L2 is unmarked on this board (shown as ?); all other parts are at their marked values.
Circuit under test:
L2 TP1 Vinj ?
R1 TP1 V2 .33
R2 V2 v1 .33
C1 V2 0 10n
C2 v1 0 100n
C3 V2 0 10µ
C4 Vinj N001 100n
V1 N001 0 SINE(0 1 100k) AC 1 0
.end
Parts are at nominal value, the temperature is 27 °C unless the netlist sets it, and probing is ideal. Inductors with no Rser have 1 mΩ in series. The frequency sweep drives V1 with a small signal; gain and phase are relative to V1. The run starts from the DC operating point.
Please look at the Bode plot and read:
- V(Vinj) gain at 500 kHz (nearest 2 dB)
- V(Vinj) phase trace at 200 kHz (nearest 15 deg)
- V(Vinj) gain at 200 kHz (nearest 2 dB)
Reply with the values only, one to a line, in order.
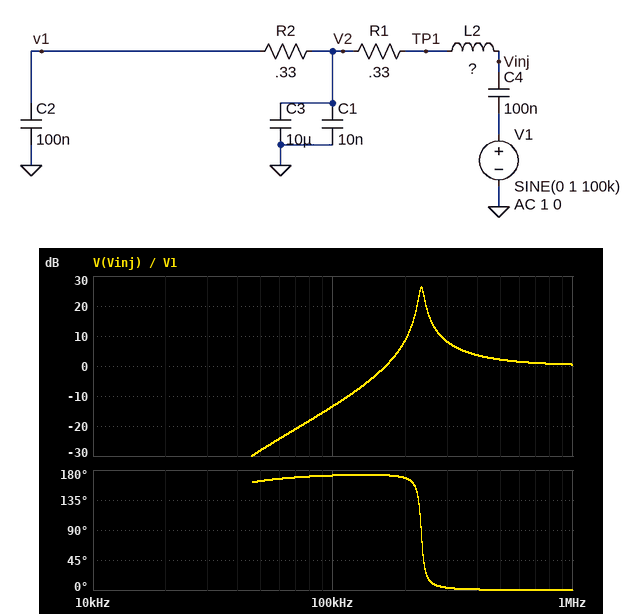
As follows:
2 dB
165 deg
8 dB
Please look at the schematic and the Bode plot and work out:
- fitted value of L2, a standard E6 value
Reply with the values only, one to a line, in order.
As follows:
4.7 µH
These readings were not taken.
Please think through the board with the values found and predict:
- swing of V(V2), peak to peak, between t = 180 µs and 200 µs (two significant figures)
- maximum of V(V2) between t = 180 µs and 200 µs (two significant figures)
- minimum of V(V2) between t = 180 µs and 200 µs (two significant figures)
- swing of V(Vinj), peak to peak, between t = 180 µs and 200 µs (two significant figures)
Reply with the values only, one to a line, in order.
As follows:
24 mV
12 mV
-12 mV
430 mV
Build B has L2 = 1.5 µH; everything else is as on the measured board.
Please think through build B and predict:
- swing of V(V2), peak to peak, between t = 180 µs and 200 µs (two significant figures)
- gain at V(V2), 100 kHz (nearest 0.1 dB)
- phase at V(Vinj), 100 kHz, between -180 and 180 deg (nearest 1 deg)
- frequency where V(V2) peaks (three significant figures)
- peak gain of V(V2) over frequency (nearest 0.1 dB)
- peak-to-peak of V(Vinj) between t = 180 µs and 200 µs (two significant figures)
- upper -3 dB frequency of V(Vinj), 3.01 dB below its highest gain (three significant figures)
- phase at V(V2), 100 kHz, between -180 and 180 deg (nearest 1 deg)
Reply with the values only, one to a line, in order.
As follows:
21 mV
-39.7 dB
156 deg
412 kHz
-18.8 dB
110 mV
433 kHz
-1 deg
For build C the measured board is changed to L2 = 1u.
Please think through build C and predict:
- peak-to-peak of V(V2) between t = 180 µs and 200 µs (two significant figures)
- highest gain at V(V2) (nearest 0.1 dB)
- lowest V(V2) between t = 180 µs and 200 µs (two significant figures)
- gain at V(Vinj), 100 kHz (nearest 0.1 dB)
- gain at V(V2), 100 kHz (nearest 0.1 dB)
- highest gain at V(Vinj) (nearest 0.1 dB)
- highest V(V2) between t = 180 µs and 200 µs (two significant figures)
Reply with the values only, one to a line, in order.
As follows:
20 mV
-20.5 dB
-10 mV
-28.6 dB
-39.8 dB
19.6 dB
10 mV
